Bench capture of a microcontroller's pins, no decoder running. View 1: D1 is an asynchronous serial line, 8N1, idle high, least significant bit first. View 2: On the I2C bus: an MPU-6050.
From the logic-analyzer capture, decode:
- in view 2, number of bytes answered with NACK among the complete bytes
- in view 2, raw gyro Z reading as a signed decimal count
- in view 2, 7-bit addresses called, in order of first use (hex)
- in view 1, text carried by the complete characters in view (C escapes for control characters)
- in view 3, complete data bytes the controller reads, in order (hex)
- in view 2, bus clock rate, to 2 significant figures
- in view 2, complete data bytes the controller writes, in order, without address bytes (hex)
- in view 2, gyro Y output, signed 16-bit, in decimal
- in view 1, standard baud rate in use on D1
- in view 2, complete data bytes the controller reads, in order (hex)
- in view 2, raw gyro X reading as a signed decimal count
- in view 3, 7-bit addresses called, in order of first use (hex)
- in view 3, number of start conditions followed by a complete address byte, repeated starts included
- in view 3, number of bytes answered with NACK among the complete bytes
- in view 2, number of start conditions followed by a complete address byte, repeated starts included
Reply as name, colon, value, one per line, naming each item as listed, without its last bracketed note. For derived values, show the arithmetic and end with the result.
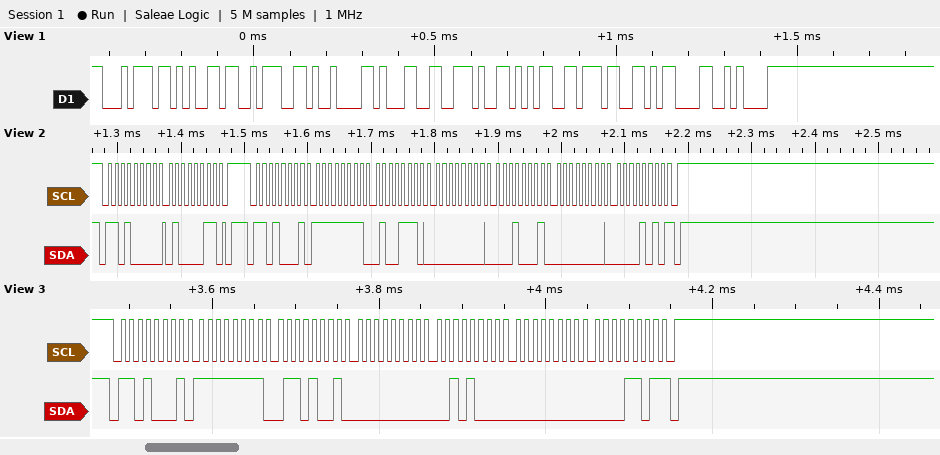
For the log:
in view 2, number of bytes answered with NACK among the complete bytes: 1
in view 2, raw gyro Z reading as a signed decimal count: 0x000A = 10
in view 2, 7-bit addresses called, in order of first use: 0x68
in view 1, text carried by the complete characters in view: "te:\t1.57\r\n"
in view 3, complete data bytes the controller reads, in order: FF 69 00 28 00 0D
in view 2, bus clock rate, to 2 significant figures: 100 kHz
in view 2, complete data bytes the controller writes, in order, without address bytes: 43
in view 2, gyro Y output, signed 16-bit, in decimal: 0x0011 = 17
in view 1, standard baud rate in use on D1: 57600 baud
in view 2, complete data bytes the controller reads, in order: FF 4E 00 11 00 0A
in view 2, raw gyro X reading as a signed decimal count: 0xFF4E = -178
in view 3, 7-bit addresses called, in order of first use: 0x68
in view 3, number of start conditions followed by a complete address byte, repeated starts included: 1
in view 3, number of bytes answered with NACK among the complete bytes: 1
in view 2, number of start conditions followed by a complete address byte, repeated starts included: 2
